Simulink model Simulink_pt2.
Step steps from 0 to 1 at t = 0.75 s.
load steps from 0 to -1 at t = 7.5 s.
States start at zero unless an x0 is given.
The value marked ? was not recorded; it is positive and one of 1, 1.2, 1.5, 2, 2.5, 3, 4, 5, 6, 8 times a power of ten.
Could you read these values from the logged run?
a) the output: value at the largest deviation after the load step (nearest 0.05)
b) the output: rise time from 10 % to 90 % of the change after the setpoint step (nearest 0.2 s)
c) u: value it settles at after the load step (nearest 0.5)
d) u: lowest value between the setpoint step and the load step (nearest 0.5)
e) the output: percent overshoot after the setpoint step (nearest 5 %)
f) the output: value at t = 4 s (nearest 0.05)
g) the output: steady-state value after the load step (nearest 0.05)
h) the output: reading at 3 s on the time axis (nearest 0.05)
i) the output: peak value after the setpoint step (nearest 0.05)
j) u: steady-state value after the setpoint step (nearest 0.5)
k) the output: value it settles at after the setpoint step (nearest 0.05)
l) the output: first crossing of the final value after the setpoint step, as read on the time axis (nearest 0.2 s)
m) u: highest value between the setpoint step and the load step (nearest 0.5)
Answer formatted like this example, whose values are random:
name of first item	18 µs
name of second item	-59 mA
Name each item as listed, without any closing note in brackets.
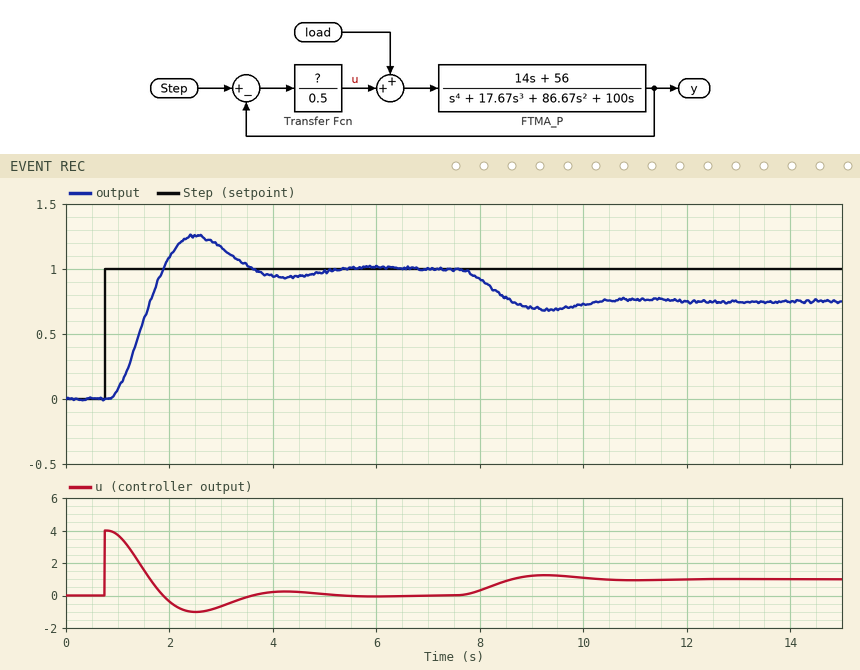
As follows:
the output: value at the largest deviation after the load step	0.70
the output: rise time from 10 % to 90 % of the change after the setpoint step	0.8 s
u: value it settles at after the load step	1.0
u: lowest value between the setpoint step and the load step	-1.0
the output: percent overshoot after the setpoint step	25 %
the output: value at t = 4 s	0.95
the output: steady-state value after the load step	0.75
the output: reading at 3 s on the time axis	1.15
the output: peak value after the setpoint step	1.25
u: steady-state value after the setpoint step	0.0
the output: value it settles at after the setpoint step	1.00
the output: first crossing of the final value after the setpoint step, as read on the time axis	1.8 s
u: highest value between the setpoint step and the load step	4.0
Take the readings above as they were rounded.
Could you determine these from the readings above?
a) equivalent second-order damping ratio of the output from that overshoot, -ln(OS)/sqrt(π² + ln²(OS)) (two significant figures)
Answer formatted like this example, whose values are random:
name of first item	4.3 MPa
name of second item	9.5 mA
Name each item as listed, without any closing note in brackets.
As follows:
equivalent second-order damping ratio of the output from that overshoot, -ln(OS)/sqrt(π² + ln²(OS))	0.40
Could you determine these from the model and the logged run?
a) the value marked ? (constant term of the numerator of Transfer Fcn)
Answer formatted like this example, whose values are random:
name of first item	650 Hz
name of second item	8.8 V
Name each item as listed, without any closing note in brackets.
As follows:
the value marked ?	2
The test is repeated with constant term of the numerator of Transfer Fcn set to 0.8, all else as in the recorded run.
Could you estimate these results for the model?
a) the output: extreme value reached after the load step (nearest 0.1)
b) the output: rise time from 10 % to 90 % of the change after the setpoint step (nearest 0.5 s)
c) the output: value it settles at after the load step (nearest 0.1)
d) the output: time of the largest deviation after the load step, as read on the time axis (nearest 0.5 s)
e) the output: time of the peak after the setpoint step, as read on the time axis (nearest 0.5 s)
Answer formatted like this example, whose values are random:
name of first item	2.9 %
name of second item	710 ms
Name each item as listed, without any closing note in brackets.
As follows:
the output: extreme value reached after the load step	0.3
the output: rise time from 10 % to 90 % of the change after the setpoint step	1.5 s
the output: value it settles at after the load step	0.4
the output: time of the largest deviation after the load step, as read on the time axis	11.0 s
the output: time of the peak after the setpoint step, as read on the time axis	4.0 s
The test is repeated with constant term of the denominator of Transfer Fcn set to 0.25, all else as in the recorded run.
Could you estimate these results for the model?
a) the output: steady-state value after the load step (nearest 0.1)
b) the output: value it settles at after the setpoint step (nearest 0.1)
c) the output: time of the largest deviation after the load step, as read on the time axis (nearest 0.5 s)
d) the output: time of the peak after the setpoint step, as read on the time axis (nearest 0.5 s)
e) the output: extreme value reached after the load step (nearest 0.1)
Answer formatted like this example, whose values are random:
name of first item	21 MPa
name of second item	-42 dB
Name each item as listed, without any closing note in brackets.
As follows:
the output: steady-state value after the load step	0.9
the output: value it settles at after the setpoint step	1.0
the output: time of the largest deviation after the load step, as read on the time axis	8.5 s
the output: time of the peak after the setpoint step, as read on the time axis	2.0 s
the output: extreme value reached after the load step	0.8
